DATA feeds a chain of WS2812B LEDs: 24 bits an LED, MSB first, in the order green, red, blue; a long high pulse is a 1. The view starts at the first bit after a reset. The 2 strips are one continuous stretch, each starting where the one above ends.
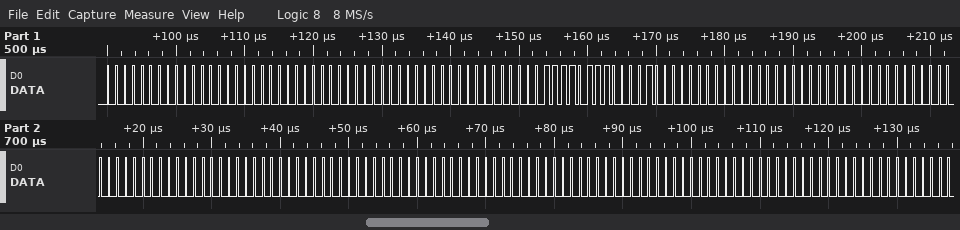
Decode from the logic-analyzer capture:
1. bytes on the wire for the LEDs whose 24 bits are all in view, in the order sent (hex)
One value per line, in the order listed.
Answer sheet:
00 00 00 00 00 00 1E E1 00 00 00 00 00 00 00 00 00 00 00 00 00 00 00 00
